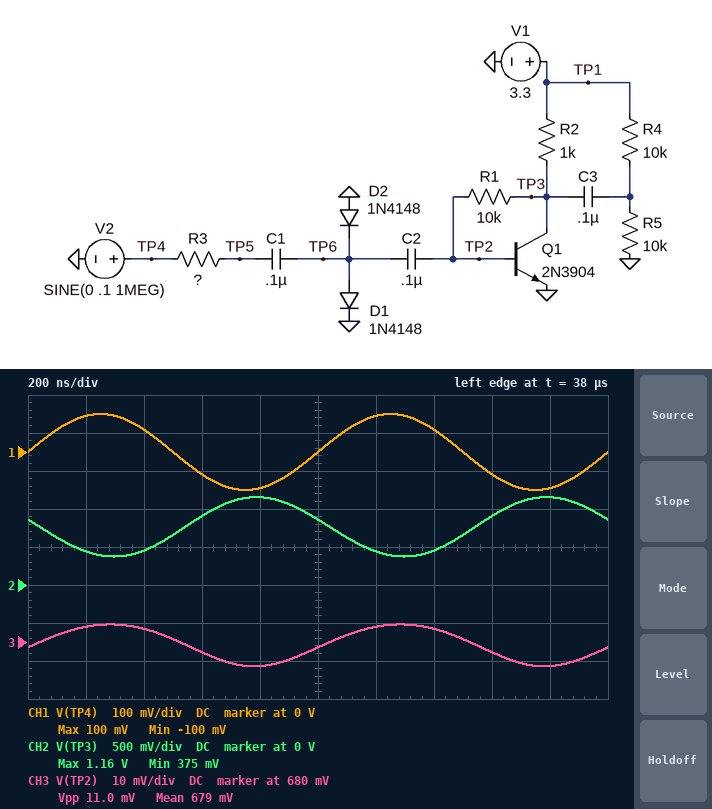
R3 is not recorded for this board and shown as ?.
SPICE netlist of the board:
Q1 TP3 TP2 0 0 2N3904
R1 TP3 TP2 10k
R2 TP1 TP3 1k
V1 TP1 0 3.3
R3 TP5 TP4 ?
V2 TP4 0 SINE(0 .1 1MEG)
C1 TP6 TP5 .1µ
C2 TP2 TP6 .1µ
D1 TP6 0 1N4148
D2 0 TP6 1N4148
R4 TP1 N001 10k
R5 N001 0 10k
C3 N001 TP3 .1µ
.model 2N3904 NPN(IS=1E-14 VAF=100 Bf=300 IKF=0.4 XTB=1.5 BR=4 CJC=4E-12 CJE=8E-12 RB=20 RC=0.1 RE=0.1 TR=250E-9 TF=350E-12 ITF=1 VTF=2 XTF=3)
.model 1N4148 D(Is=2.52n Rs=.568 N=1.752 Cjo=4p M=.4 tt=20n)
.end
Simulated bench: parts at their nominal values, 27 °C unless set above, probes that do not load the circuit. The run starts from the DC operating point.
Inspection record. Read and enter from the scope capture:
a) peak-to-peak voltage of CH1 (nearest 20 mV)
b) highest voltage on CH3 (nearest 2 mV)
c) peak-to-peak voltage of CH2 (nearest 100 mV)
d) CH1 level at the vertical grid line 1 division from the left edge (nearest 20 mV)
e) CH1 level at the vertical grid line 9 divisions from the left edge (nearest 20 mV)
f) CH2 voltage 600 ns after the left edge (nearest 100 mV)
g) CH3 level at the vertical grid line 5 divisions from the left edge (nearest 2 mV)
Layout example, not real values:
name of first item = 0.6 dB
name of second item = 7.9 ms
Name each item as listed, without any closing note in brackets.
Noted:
peak-to-peak voltage of CH1 = 200 mV
highest voltage on CH3 = 684 mV
peak-to-peak voltage of CH2 = 800 mV
CH1 level at the vertical grid line 1 division from the left edge = 100 mV
CH1 level at the vertical grid line 9 divisions from the left edge = -100 mV
CH2 voltage 600 ns after the left edge = 900 mV
CH3 level at the vertical grid line 5 divisions from the left edge = 678 mV
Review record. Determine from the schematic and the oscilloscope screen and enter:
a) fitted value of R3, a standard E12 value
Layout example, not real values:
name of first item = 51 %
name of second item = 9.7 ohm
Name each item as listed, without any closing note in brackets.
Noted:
fitted value of R3, a standard E12 value = 2.2 kΩ
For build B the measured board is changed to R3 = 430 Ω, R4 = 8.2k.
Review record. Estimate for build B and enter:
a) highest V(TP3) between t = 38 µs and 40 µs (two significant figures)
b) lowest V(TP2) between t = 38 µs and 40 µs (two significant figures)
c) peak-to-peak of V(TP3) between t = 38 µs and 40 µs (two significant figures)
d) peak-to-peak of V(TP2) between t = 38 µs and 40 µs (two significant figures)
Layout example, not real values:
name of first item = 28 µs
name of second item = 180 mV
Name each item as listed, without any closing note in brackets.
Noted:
highest V(TP3) between t = 38 µs and 40 µs = 2.2 V
lowest V(TP2) between t = 38 µs and 40 µs = 640 mV
peak-to-peak of V(TP3) between t = 38 µs and 40 µs = 2.1 V
peak-to-peak of V(TP2) between t = 38 µs and 40 µs = 49 mV
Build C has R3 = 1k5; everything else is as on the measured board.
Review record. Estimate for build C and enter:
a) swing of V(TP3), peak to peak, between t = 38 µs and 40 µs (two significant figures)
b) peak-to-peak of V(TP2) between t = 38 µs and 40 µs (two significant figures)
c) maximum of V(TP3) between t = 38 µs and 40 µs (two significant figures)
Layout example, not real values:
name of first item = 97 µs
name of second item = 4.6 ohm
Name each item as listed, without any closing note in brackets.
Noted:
swing of V(TP3), peak to peak, between t = 38 µs and 40 µs = 1.1 V
peak-to-peak of V(TP2) between t = 38 µs and 40 µs = 16 mV
maximum of V(TP3) between t = 38 µs and 40 µs = 1.3 V
